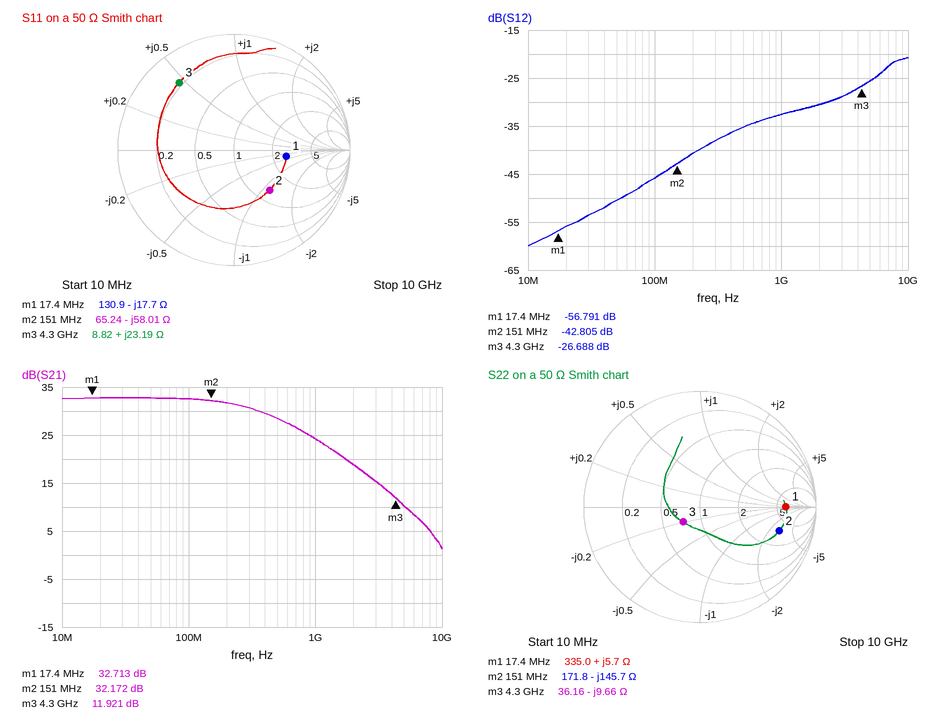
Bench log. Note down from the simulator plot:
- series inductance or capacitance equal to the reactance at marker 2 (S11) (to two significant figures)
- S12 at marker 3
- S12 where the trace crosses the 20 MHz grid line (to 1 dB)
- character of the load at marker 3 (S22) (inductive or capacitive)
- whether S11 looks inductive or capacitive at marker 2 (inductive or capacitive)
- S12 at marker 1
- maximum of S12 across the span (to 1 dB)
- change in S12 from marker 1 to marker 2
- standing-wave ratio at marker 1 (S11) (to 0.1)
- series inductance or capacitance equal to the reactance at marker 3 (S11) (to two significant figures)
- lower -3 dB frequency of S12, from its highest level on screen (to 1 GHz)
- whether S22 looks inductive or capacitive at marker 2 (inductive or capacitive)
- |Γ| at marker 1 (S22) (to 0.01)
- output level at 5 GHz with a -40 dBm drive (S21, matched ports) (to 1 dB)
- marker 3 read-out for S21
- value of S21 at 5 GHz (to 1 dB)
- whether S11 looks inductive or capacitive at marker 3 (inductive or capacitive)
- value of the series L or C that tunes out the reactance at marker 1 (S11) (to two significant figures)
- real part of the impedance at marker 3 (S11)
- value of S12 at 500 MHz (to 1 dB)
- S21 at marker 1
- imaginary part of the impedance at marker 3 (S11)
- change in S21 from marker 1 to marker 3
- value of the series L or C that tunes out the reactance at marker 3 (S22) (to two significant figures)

18 pF
-26.688 dB
-56 dB
capacitive
capacitive
-56.791 dB
-21 dB
13.986 dB
2.7
860 pH
6 GHz
capacitive
0.74
-30 dBm
11.921 dB
10 dB
inductive
160 nH
8.82 Ω
-35 dB
32.713 dB
+23.19 Ω
-20.792 dB
360 pH
